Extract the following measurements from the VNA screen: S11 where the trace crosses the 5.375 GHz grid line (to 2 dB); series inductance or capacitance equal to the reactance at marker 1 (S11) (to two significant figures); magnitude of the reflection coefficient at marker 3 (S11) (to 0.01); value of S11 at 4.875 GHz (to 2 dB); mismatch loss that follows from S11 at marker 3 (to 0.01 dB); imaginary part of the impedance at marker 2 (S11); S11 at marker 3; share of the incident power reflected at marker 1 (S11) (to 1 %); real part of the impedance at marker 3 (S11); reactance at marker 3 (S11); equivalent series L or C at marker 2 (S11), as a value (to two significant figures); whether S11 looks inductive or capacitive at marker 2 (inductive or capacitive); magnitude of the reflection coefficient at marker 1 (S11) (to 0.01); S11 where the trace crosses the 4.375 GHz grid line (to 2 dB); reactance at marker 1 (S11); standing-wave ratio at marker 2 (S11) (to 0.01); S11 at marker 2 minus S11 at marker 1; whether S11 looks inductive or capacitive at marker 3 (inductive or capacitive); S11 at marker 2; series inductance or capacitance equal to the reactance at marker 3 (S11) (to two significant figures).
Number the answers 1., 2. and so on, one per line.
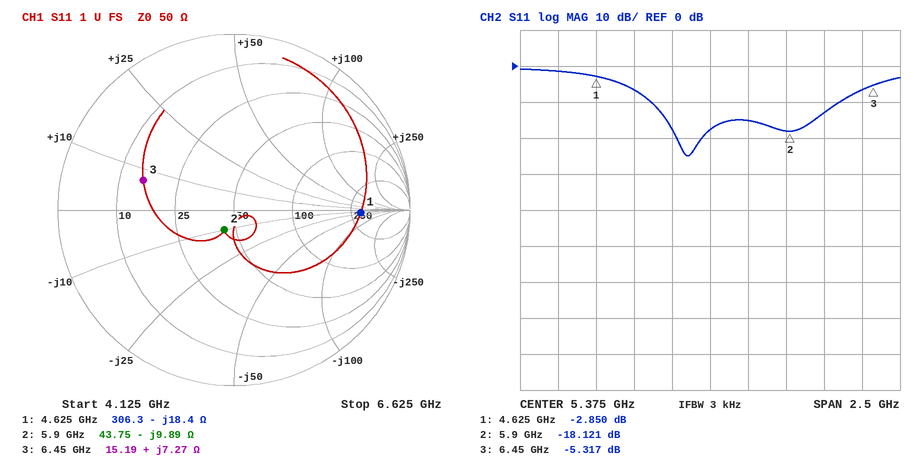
1. -18 dB
2. 1.9 pF
3. 0.54
4. -6 dB
5. 1.51 dB
6. -9.89 Ω
7. -5.317 dB
8. 52 %
9. 15.19 Ω
10. +7.27 Ω
11. 2.7 pF
12. capacitive
13. 0.72
14. -2 dB
15. -18.4 Ω
16. 1.28
17. -15.271 dB
18. inductive
19. -18.121 dB
20. 180 pH
